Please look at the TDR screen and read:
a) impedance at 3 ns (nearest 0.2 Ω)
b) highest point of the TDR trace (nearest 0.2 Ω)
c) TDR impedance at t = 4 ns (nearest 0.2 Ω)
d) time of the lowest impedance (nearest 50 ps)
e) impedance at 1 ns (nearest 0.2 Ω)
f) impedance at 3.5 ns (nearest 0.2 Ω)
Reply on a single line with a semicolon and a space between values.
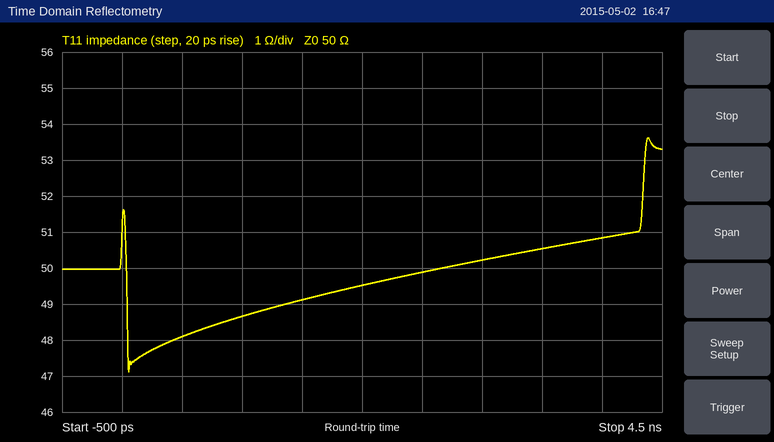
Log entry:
50.2 Ω; 53.6 Ω; 50.8 Ω; 50 ps; 48.6 Ω; 50.6 Ω
